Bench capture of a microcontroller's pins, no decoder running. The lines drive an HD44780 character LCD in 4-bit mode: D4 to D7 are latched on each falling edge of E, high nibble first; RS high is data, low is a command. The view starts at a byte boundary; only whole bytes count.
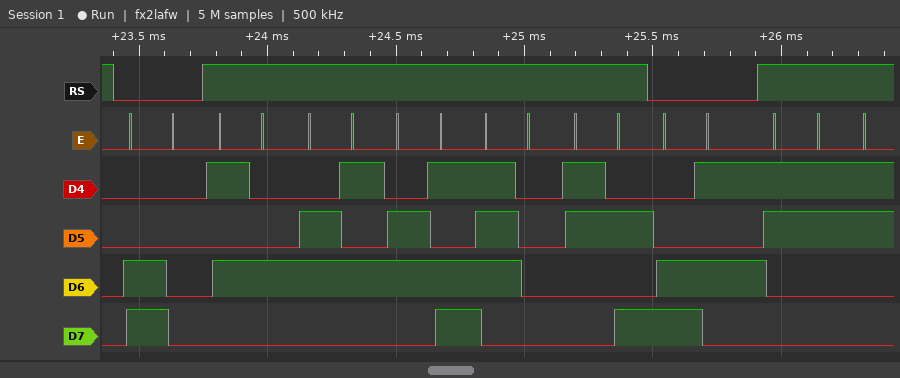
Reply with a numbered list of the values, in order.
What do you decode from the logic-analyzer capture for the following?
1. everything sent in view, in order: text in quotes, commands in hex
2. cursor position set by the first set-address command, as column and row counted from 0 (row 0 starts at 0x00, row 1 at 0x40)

1. 0xC0 "Temp:" 0xC5 "3"
2. column 0, row 1
